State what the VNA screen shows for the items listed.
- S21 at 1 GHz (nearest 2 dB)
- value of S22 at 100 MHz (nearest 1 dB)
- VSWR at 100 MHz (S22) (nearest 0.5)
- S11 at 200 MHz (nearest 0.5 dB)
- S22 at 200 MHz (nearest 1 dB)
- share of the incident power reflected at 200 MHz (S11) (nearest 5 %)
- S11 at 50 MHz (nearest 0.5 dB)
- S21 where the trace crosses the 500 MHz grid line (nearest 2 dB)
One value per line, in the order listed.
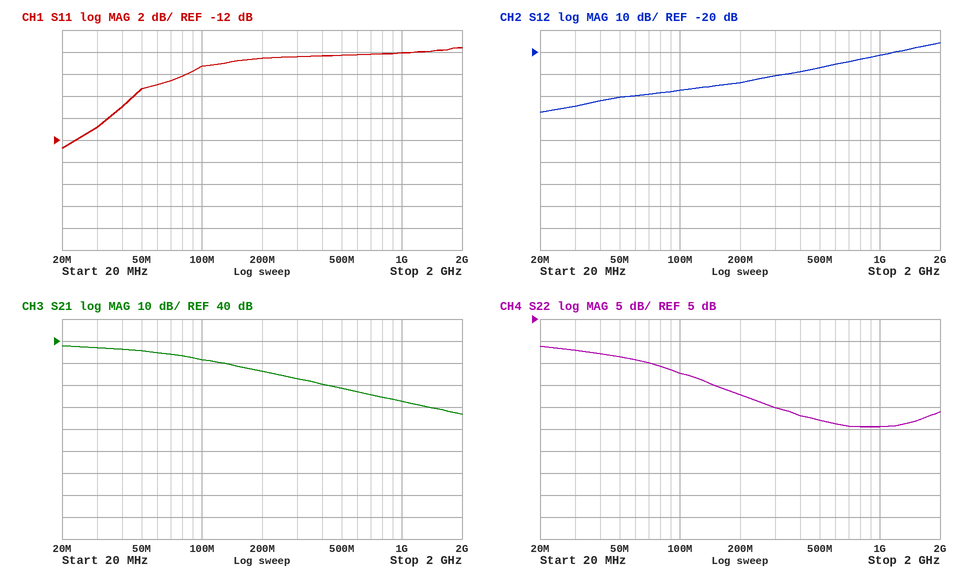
12 dB
-7 dB
2.5
-4.5 dB
-12 dB
35 %
-7.5 dB
18 dB
